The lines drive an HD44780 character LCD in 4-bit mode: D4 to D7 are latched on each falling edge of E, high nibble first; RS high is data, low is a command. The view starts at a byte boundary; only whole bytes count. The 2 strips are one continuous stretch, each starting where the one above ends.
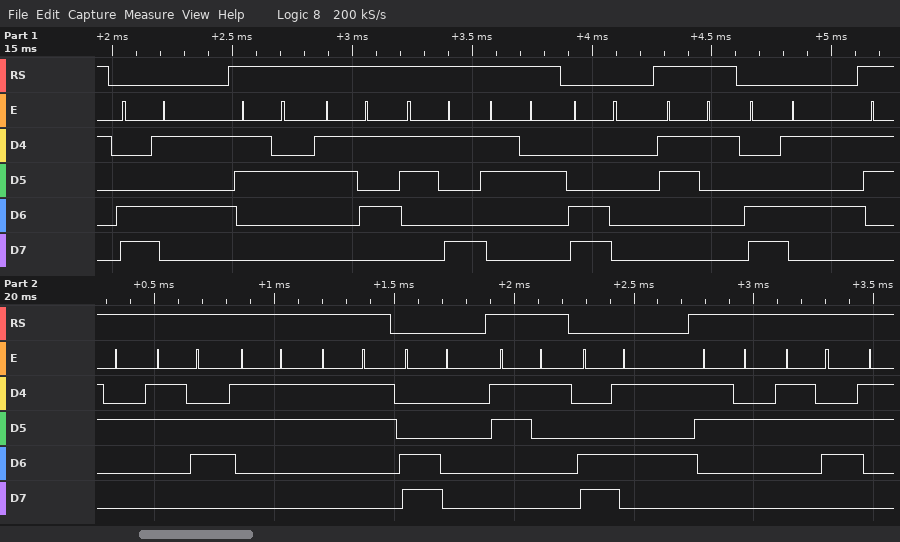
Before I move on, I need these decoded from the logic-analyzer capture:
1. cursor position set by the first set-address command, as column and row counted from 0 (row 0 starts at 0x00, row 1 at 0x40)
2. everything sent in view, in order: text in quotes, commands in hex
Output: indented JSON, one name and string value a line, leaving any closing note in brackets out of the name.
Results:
{
  "cursor position set by the first set-address command, as column and row counted from 0": "column 5, row 1",
  "everything sent in view, in order: text in quotes, commands in hex": "0xC5 \"2592\" 0xC0 \"1\" 0xC5 \"2633\" 0xC0 \"1\" 0xC5 \"26\""
}
